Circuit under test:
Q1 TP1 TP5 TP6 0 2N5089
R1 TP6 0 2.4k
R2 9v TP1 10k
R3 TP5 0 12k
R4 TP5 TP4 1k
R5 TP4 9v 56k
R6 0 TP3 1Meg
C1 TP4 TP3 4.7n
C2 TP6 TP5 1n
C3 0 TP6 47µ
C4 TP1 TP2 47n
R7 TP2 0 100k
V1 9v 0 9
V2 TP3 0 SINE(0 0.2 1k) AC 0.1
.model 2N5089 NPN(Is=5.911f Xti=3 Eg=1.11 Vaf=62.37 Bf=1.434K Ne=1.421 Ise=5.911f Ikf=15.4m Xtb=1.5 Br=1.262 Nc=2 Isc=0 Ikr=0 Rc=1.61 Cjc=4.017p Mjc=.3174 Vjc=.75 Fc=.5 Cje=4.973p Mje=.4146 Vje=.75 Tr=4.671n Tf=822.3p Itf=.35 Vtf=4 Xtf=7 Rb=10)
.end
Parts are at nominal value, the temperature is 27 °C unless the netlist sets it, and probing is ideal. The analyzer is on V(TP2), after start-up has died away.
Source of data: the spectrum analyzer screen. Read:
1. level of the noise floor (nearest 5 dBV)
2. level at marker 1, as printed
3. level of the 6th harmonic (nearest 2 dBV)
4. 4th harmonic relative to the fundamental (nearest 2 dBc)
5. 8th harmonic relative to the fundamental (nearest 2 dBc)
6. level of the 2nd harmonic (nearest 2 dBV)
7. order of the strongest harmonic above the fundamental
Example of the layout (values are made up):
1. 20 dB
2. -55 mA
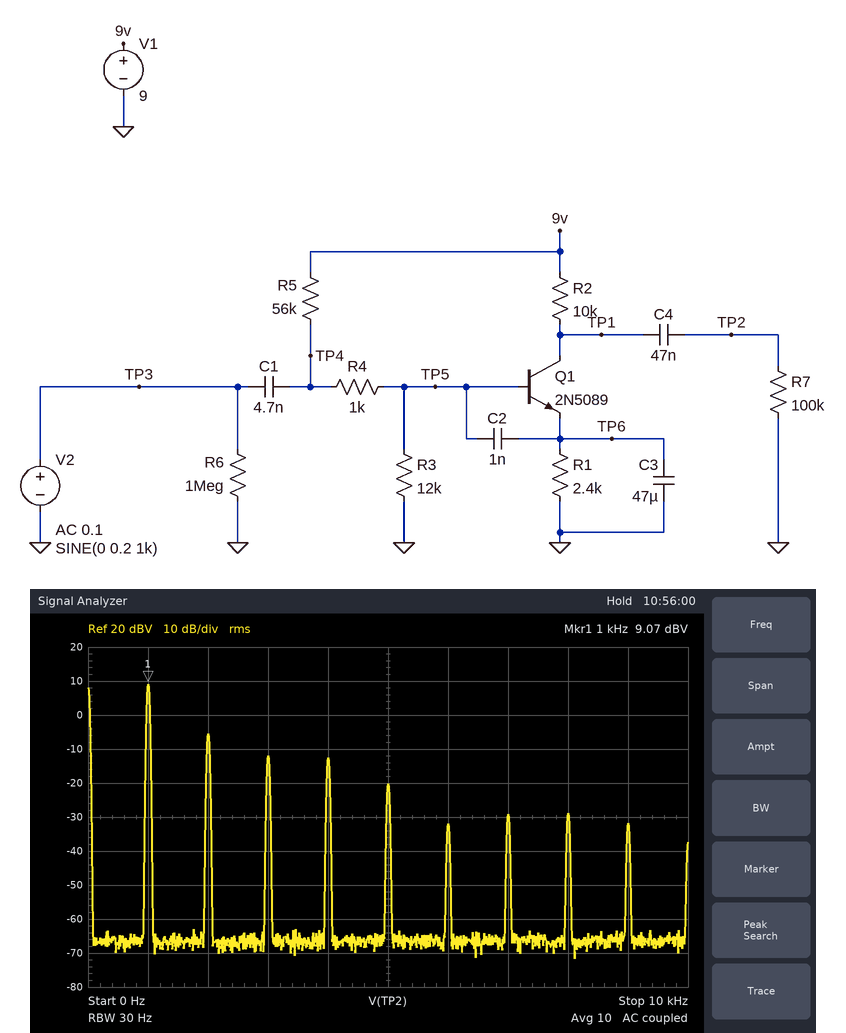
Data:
1. -65 dBV
2. 9.07 dBV
3. -32 dBV
4. -22 dBc
5. -38 dBc
6. -6 dBV
7. 2
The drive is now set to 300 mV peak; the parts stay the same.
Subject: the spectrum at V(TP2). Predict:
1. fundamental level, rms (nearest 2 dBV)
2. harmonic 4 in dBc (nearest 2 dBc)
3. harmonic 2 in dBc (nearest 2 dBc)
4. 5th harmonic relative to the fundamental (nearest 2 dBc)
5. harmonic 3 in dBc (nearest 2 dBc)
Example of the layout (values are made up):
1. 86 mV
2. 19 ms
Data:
1. 10 dBV
2. -20 dBc
3. -16 dBc
4. -34 dBc
5. -16 dBc
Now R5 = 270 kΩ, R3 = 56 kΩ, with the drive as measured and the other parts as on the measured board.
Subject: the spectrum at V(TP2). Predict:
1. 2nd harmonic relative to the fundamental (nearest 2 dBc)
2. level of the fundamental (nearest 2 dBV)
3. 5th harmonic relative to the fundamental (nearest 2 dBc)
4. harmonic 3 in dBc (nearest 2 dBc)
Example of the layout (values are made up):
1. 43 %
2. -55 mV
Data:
1. -14 dBc
2. 10 dBV
3. -28 dBc
4. -14 dBc
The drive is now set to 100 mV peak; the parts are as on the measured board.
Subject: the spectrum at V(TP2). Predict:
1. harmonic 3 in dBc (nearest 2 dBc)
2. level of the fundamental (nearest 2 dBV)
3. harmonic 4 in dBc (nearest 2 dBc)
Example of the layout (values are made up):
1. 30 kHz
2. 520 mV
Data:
1. -40 dBc
2. 6 dBV
3. -56 dBc
